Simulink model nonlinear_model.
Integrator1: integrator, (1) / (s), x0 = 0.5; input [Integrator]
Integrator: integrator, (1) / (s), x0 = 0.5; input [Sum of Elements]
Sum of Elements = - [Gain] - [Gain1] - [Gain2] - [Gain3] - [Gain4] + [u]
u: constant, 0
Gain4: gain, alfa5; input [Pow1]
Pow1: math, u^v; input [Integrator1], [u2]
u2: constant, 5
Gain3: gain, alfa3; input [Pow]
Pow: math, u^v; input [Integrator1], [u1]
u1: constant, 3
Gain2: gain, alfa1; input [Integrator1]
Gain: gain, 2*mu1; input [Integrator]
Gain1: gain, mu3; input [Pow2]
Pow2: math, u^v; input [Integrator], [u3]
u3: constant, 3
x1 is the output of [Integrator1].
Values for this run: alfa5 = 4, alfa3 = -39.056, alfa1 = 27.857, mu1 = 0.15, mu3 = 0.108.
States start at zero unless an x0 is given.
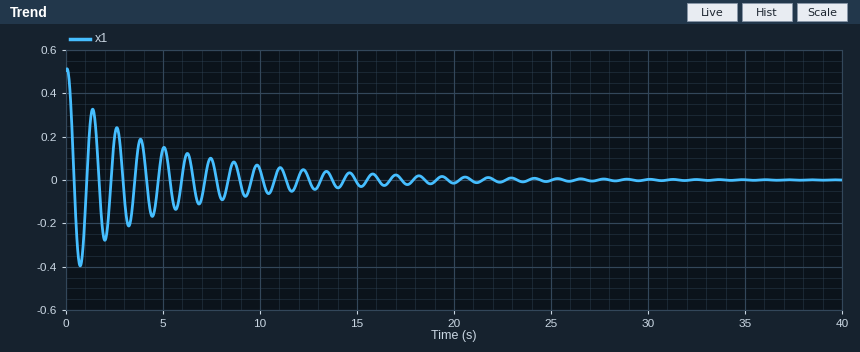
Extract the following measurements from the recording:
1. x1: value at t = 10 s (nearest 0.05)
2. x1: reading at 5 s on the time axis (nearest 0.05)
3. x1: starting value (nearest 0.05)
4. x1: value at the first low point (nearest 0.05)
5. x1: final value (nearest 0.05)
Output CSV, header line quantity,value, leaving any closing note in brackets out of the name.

quantity,value
x1: value at t = 10 s,0.05
x1: reading at 5 s on the time axis,0.15
x1: starting value,0.50
x1: value at the first low point,-0.40
x1: final value,0.00
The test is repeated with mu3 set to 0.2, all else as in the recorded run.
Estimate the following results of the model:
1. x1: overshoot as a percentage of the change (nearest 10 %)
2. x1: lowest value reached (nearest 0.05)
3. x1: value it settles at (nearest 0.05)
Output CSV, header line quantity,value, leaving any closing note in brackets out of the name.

quantity,value
x1: overshoot as a percentage of the change,70 %
x1: lowest value reached,-0.35
x1: value it settles at,0.00
